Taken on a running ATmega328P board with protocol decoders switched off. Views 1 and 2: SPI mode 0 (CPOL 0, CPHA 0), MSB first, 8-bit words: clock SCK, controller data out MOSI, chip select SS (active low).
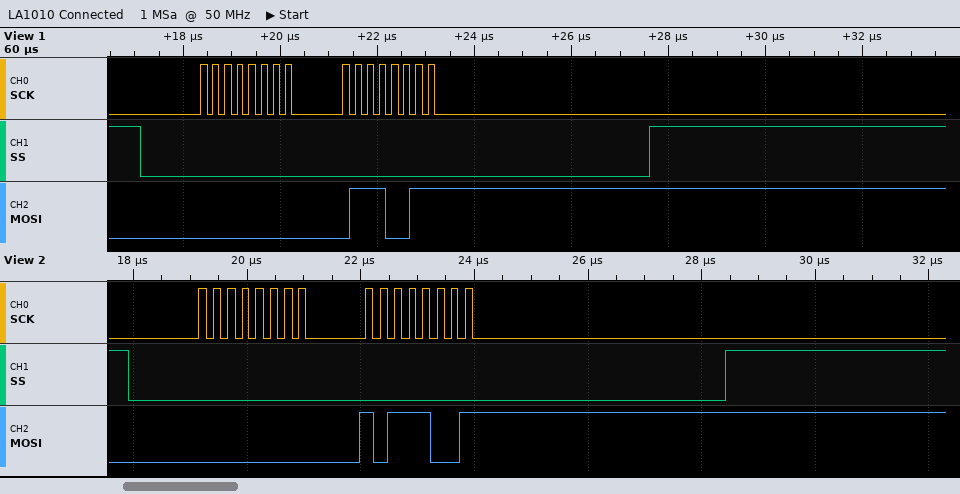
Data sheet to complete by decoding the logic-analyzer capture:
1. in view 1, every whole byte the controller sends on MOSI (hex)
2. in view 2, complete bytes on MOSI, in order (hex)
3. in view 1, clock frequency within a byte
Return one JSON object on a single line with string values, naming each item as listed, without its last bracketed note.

{"in view 1, every whole byte the controller sends on MOSI": "0x00 0x73", "in view 2, complete bytes on MOSI, in order": "00 B9", "in view 1, clock frequency within a byte": "4 MHz"}
